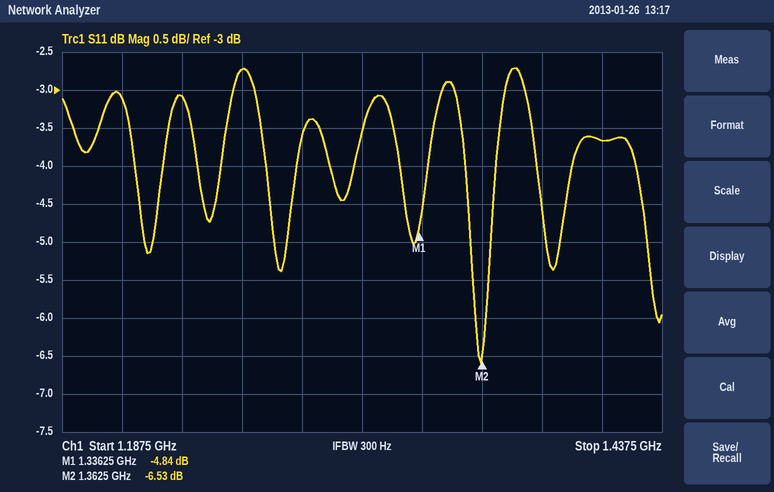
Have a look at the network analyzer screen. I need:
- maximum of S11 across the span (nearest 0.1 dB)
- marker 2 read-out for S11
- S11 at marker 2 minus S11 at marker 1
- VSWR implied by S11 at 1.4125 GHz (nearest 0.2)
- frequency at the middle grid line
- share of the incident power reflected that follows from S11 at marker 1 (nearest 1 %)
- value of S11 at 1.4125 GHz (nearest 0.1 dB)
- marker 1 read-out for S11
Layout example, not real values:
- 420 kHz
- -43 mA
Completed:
- -2.7 dB
- -6.53 dB
- -1.69 dB
- 4.8
- 1.3125 GHz
- 33 %
- -3.7 dB
- -4.84 dB
